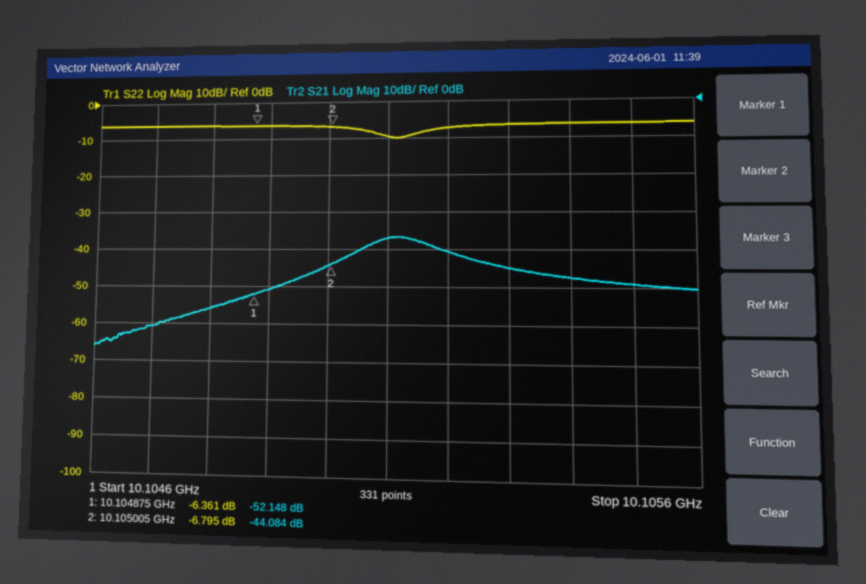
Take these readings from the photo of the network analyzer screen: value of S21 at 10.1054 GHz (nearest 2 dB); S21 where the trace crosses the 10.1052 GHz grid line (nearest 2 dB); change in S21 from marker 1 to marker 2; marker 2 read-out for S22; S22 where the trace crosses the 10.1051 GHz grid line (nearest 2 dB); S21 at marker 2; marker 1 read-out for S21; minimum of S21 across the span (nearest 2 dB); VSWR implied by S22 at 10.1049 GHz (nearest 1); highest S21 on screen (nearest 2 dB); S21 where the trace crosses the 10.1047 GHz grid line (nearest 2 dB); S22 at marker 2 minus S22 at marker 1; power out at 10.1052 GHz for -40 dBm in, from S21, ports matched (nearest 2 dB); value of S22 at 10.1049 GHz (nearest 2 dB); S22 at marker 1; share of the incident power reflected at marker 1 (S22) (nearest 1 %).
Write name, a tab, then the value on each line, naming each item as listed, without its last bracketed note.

value of S21 at 10.1054 GHz	-48 dB
S21 where the trace crosses the 10.1052 GHz grid line	-40 dB
change in S21 from marker 1 to marker 2	8.064 dB
marker 2 read-out for S22	-6.795 dB
S22 where the trace crosses the 10.1051 GHz grid line	-10 dB
S21 at marker 2	-44.084 dB
marker 1 read-out for S21	-52.148 dB
minimum of S21 across the span	-66 dB
VSWR implied by S22 at 10.1049 GHz	3
highest S21 on screen	-36 dB
S21 where the trace crosses the 10.1047 GHz grid line	-60 dB
S22 at marker 2 minus S22 at marker 1	-0.434 dB
power out at 10.1052 GHz for -40 dBm in, from S21, ports matched	-80 dBm
value of S22 at 10.1049 GHz	-6 dB
S22 at marker 1	-6.361 dB
share of the incident power reflected at marker 1 (S22)	23 %
